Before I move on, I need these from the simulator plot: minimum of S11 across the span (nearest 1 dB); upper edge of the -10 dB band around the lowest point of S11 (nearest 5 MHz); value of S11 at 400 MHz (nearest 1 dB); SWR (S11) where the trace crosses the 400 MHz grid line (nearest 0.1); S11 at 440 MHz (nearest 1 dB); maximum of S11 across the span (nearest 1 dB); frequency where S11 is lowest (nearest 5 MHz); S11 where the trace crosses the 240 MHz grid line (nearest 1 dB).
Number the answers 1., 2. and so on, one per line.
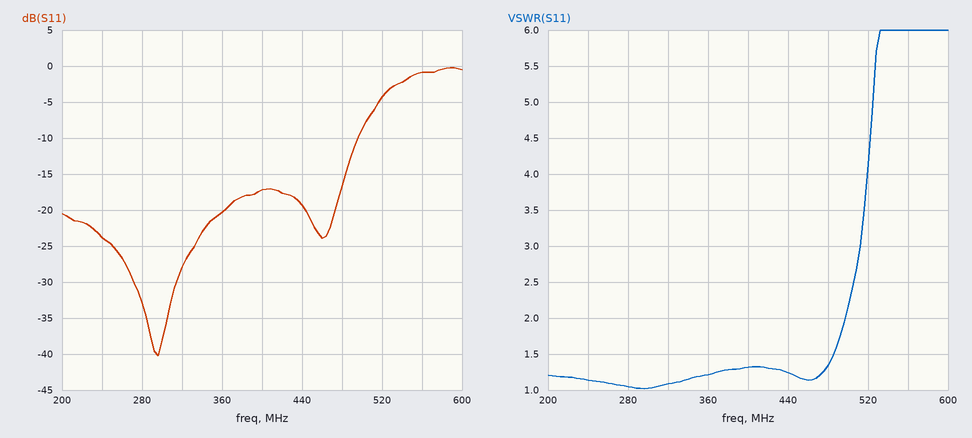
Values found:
1. -40 dB
2. 495 MHz
3. -17 dB
4. 1.3
5. -19 dB
6. 0 dB
7. 295 MHz
8. -24 dB
